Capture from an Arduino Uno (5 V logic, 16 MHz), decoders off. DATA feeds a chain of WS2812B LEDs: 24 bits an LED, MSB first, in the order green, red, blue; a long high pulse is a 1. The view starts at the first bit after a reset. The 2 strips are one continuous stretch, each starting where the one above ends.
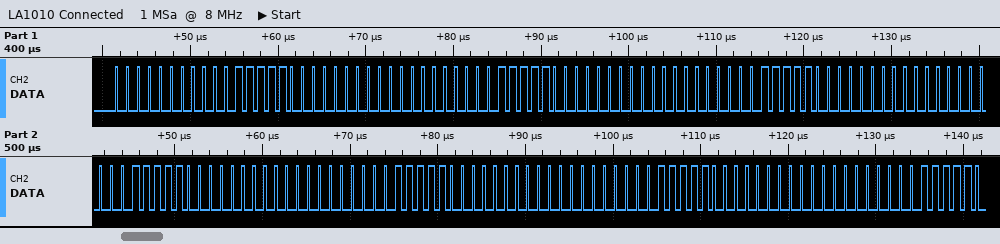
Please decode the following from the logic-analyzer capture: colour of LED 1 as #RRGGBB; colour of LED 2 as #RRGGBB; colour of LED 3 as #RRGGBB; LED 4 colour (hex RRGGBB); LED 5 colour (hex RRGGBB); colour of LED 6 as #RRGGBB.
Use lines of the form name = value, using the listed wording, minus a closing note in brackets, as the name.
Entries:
colour of LED 1 as #RRGGBB = #1F0000
colour of LED 2 as #RRGGBB = #1F0000
colour of LED 3 as #RRGGBB = #1F0000
LED 4 colour = #1F0000
LED 5 colour = #1F0000
colour of LED 6 as #RRGGBB = #1F0000
